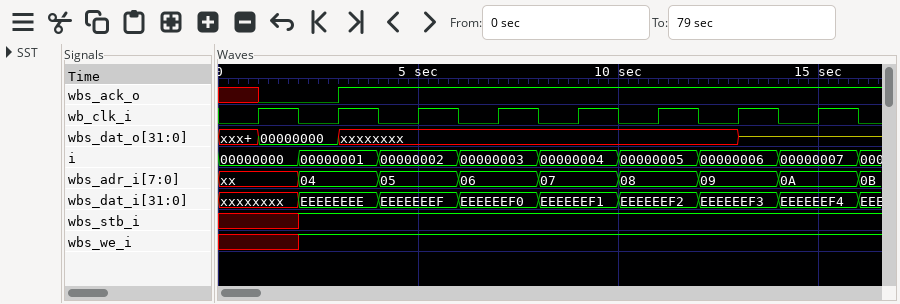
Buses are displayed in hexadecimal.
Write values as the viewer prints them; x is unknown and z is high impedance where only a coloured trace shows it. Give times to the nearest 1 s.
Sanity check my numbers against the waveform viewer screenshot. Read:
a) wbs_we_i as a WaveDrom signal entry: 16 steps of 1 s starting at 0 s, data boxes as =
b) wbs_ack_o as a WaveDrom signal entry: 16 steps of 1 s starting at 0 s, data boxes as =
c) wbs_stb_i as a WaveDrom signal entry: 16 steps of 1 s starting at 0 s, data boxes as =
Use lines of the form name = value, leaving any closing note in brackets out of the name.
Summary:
wbs_we_i as a WaveDrom signal entry: 16 steps of 1 s starting at 0 s, data boxes as = = {name: 'wbs_we_i', wave: 'x.1.............'}
wbs_ack_o as a WaveDrom signal entry: 16 steps of 1 s starting at 0 s, data boxes as = = {name: 'wbs_ack_o', wave: 'x0.1............'}
wbs_stb_i as a WaveDrom signal entry: 16 steps of 1 s starting at 0 s, data boxes as = = {name: 'wbs_stb_i', wave: 'x.1.............'}
